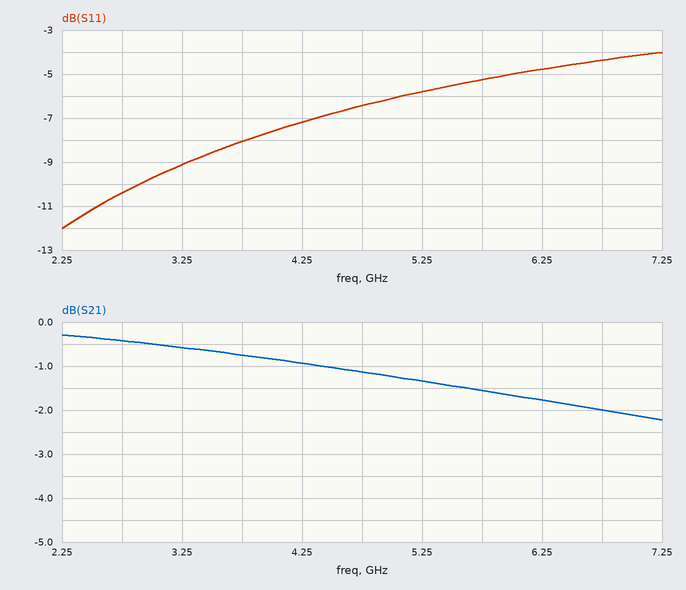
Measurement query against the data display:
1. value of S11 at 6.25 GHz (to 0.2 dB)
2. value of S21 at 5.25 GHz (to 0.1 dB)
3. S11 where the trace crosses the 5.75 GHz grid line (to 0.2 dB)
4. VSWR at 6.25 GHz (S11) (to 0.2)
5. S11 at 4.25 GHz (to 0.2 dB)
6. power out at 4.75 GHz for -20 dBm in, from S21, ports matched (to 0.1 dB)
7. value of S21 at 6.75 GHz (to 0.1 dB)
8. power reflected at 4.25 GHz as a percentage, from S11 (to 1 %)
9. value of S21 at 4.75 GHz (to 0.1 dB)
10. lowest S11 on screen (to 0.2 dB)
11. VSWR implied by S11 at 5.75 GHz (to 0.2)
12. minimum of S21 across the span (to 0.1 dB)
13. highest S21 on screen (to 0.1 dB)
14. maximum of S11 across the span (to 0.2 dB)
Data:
-4.8 dB
-1.3 dB
-5.2 dB
3.8
-7.2 dB
-21.1 dBm
-2.0 dB
19 %
-1.1 dB
-12.0 dB
3.4
-2.2 dB
-0.3 dB
-4.0 dB
